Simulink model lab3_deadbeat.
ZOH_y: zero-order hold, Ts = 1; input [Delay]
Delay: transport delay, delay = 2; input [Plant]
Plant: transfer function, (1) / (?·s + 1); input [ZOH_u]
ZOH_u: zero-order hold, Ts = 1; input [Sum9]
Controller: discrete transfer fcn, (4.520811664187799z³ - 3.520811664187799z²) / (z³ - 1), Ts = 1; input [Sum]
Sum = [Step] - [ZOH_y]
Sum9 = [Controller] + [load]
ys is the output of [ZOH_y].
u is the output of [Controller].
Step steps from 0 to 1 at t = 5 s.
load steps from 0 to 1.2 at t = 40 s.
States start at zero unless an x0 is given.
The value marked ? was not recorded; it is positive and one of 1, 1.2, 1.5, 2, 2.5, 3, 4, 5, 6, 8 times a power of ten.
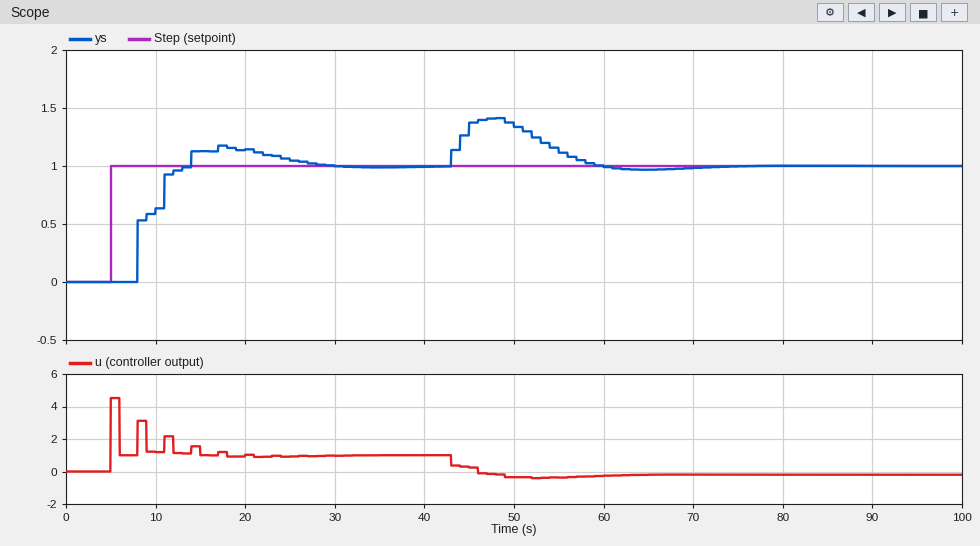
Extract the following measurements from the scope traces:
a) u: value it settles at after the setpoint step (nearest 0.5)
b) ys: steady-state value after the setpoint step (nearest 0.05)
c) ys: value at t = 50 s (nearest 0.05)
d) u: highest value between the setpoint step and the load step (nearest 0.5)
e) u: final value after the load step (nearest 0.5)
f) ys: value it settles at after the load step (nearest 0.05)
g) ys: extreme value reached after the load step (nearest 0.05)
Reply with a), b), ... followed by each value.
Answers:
a) 1.0
b) 1.00
c) 1.35
d) 4.5
e) 0.0
f) 1.00
g) 1.40
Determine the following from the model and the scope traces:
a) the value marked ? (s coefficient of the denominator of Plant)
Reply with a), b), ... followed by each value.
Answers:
a) 8
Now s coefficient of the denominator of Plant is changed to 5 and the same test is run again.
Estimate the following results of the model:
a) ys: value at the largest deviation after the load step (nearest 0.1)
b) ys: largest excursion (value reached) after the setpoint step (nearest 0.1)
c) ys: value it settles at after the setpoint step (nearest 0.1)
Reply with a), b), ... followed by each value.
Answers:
a) 1.5
b) 1.1
c) 1.0
